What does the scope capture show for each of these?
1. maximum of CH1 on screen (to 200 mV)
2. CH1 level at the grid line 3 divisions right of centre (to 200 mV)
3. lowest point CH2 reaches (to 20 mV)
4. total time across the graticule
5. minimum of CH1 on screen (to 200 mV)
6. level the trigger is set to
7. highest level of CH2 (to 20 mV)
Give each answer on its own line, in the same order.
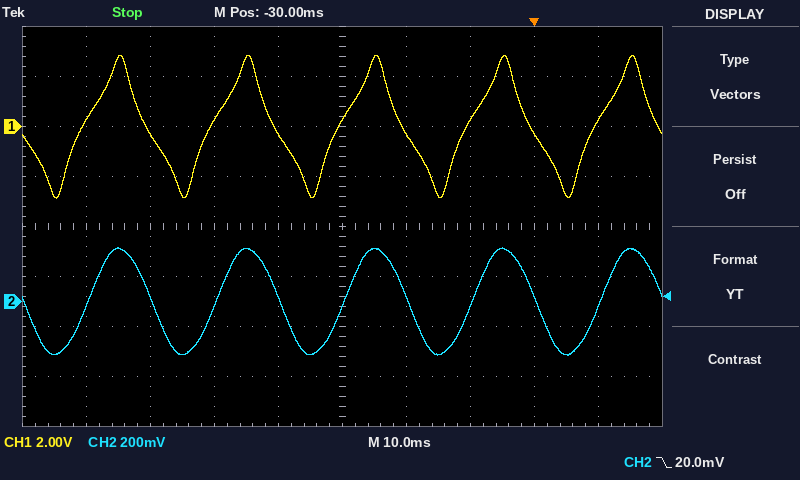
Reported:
2.8 V
-200 mV
-220 mV
100 ms
-2.8 V
20.0 mV
220 mV
